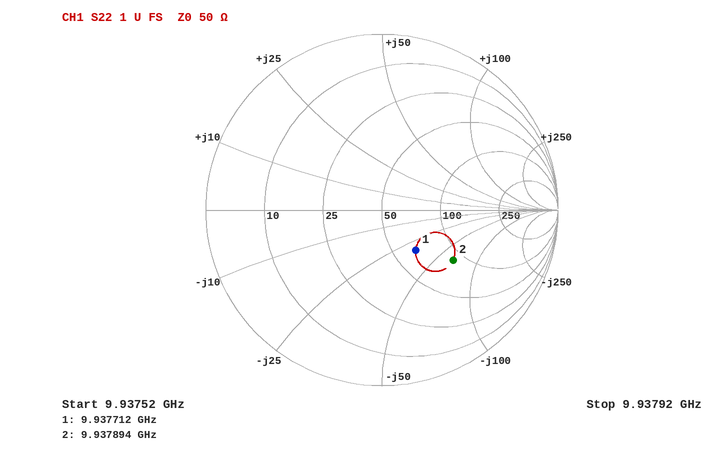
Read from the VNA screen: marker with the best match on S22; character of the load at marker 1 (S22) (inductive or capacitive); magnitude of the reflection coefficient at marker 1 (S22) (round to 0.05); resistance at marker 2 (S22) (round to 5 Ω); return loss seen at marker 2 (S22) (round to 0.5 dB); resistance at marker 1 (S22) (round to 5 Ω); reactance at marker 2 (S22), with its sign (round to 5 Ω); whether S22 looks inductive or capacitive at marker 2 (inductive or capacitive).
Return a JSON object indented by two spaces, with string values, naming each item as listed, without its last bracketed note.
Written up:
{
  "marker with the best match on S22": "marker 1",
  "character of the load at marker 1 (S22)": "capacitive",
  "magnitude of the reflection coefficient at marker 1 (S22)": "0.30",
  "resistance at marker 2 (S22)": "85 Ω",
  "return loss seen at marker 2 (S22)": "6.0 dB",
  "resistance at marker 1 (S22)": "65 Ω",
  "reactance at marker 2 (S22), with its sign": "-65 Ω",
  "whether S22 looks inductive or capacitive at marker 2": "capacitive"
}
